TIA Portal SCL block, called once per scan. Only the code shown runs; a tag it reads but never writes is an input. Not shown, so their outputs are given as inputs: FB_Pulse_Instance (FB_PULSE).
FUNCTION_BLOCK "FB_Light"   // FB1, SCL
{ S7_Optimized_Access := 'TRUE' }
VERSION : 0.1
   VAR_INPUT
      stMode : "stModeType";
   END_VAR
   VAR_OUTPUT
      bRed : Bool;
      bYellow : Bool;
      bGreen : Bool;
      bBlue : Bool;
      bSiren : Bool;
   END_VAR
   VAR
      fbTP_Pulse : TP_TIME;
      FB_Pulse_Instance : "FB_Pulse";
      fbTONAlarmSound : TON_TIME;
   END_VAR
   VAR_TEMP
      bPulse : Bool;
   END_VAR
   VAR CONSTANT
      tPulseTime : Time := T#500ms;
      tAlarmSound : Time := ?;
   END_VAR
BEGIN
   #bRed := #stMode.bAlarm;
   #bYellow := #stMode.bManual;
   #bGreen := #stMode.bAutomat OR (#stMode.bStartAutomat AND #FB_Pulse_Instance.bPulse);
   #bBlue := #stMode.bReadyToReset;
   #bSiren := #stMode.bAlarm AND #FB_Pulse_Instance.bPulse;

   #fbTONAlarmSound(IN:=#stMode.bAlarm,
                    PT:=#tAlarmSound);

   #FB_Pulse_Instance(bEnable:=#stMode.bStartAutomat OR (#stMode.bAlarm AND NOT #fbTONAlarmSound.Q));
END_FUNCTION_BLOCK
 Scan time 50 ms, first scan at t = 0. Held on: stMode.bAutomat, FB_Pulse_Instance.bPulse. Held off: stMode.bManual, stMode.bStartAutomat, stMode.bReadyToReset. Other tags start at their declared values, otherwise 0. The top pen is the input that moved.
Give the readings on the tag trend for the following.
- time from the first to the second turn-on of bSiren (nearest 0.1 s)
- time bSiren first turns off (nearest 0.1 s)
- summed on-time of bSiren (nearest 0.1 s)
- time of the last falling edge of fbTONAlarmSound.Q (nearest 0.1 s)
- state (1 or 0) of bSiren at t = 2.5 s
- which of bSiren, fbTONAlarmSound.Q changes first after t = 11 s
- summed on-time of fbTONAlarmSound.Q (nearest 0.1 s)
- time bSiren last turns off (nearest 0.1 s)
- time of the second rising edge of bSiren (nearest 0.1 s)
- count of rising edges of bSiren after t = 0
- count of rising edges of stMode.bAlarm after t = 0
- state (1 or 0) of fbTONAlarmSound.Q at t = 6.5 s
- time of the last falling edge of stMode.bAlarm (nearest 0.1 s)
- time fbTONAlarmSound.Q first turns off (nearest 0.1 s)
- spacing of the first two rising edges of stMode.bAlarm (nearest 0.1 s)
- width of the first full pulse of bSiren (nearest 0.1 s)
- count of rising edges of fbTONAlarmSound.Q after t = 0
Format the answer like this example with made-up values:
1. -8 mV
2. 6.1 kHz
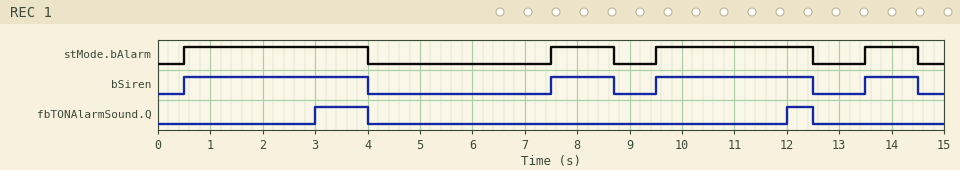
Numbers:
1. 7.0 s
2. 4.0 s
3. 8.7 s
4. 12.5 s
5. 1
6. fbTONAlarmSound.Q
7. 1.5 s
8. 14.5 s
9. 7.5 s
10. 4
11. 4
12. 0
13. 14.5 s
14. 4.0 s
15. 7.0 s
16. 3.5 s
17. 2
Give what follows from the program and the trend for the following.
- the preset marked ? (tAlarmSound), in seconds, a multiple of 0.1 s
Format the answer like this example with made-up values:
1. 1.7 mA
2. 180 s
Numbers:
1. 2.5 s
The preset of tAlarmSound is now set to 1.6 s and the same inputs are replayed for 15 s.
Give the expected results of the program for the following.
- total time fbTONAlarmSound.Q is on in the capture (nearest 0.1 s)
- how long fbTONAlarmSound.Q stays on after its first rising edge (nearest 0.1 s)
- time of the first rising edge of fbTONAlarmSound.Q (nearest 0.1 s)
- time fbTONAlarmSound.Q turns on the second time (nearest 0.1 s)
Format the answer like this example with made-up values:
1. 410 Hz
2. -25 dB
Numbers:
1. 3.3 s
2. 1.9 s
3. 2.1 s
4. 11.1 s
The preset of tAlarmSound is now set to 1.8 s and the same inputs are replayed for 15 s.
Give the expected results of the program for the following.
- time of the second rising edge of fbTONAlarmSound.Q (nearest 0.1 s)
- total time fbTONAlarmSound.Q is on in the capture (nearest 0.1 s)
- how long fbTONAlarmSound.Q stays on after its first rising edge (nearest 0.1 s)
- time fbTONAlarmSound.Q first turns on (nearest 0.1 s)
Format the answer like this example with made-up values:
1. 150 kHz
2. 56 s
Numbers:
1. 11.3 s
2. 2.9 s
3. 1.7 s
4. 2.3 s
